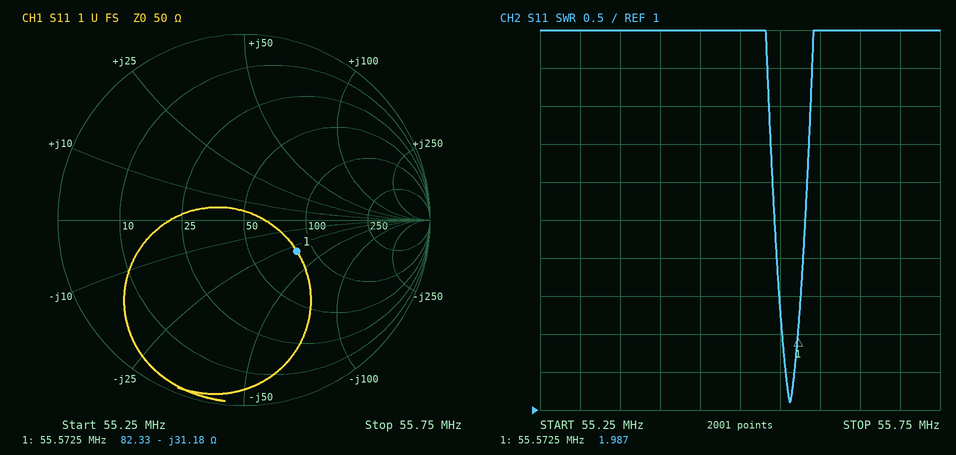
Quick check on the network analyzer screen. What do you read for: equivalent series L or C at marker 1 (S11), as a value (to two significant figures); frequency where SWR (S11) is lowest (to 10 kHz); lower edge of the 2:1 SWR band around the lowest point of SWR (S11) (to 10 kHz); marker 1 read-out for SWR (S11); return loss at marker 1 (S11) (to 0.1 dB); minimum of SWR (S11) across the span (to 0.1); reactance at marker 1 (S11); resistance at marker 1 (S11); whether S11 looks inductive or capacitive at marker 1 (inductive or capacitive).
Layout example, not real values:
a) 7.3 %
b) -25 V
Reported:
a) 92 pF
b) 55.56 MHz
c) 55.55 MHz
d) 1.987
e) 9.6 dB
f) 1.1
g) -31.18 Ω
h) 82.33 Ω
i) capacitive
